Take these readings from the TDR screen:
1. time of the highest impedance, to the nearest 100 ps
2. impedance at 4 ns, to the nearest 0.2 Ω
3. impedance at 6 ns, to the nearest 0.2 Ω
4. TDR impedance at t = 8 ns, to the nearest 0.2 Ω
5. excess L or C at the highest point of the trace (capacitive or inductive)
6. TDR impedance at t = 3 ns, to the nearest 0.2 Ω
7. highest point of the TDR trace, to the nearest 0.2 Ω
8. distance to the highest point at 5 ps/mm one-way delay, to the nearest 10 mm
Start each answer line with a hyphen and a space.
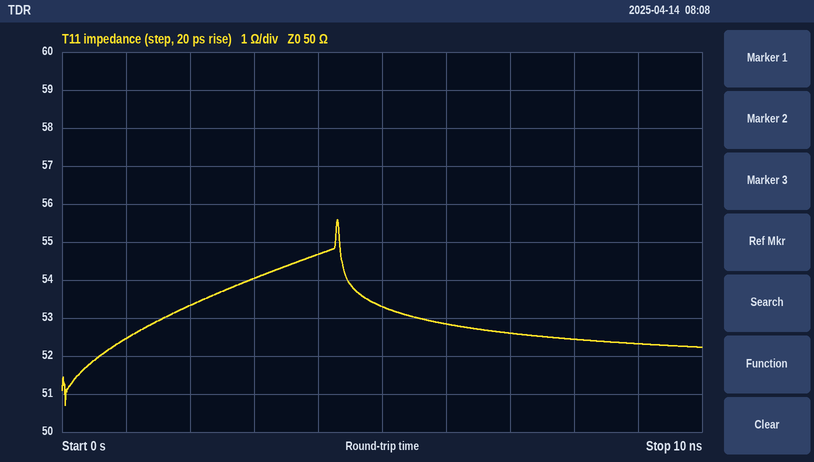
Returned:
- 4.3 ns
- 54.6 Ω
- 52.8 Ω
- 52.4 Ω
- inductive
- 54.0 Ω
- 55.6 Ω
- 430 mm
